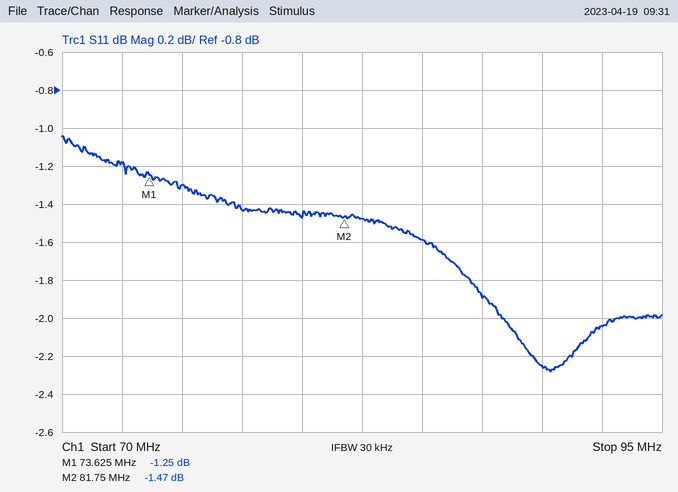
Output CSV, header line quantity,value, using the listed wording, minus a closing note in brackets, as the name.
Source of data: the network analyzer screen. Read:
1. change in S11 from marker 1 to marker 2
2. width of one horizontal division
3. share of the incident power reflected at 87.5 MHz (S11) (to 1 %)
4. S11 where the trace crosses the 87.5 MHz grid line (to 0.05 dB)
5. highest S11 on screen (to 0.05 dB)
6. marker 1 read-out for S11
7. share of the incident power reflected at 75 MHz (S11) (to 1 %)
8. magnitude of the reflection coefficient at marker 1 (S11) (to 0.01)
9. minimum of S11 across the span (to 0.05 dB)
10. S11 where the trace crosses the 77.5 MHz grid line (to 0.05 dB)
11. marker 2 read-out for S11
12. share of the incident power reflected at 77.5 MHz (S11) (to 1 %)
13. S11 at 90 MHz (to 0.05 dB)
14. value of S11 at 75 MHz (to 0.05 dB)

quantity,value
change in S11 from marker 1 to marker 2,-0.22 dB
width of one horizontal division,2.5 MHz
share of the incident power reflected at 87.5 MHz (S11),65 %
S11 where the trace crosses the 87.5 MHz grid line,-1.90 dB
highest S11 on screen,-1.05 dB
marker 1 read-out for S11,-1.25 dB
share of the incident power reflected at 75 MHz (S11),74 %
magnitude of the reflection coefficient at marker 1 (S11),0.87
minimum of S11 across the span,-2.30 dB
S11 where the trace crosses the 77.5 MHz grid line,-1.45 dB
marker 2 read-out for S11,-1.47 dB
share of the incident power reflected at 77.5 MHz (S11),72 %
S11 at 90 MHz,-2.25 dB
value of S11 at 75 MHz,-1.30 dB
